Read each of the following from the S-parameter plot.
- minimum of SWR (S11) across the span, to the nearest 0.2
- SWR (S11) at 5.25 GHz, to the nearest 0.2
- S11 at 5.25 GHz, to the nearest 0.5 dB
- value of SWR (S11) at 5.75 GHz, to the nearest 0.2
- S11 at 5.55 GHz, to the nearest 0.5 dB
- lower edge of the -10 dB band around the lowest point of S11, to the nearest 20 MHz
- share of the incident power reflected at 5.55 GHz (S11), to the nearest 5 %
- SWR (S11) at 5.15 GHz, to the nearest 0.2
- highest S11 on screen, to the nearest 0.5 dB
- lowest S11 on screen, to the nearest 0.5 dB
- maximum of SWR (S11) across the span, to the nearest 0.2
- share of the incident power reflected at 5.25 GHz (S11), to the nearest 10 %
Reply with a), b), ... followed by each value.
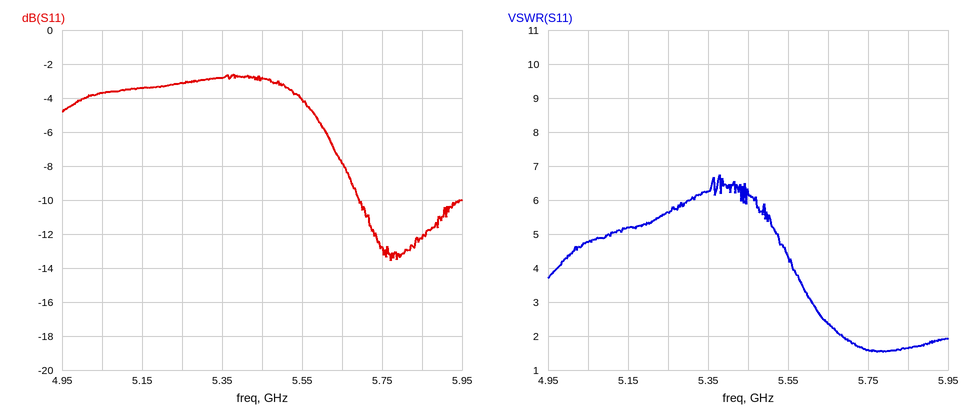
a) 1.6
b) 5.6
c) -3.0 dB
d) 1.6
e) -4.0 dB
f) 5.70 GHz
g) 40 %
h) 5.2
i) -2.5 dB
j) -13.5 dB
k) 6.8
l) 50 %
